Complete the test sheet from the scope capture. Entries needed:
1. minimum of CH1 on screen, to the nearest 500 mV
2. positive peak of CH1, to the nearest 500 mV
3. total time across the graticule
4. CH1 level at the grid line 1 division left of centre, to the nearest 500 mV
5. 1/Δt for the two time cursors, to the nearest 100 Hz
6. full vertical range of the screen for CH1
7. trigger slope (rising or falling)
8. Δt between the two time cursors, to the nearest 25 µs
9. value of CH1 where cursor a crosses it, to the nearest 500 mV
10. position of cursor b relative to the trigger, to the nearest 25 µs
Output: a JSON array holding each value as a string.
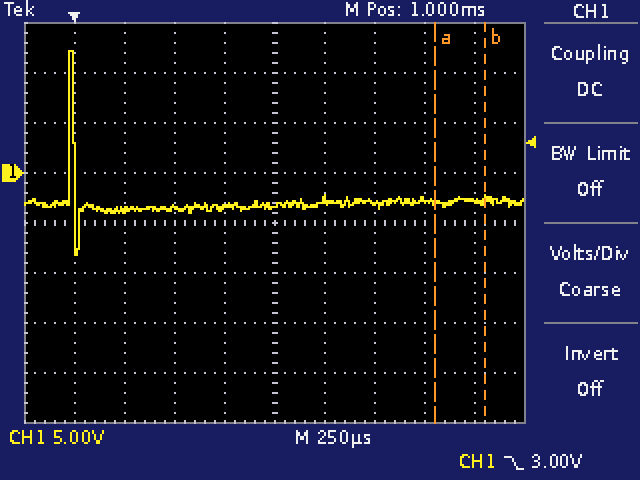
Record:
["-8.0 V", "12.0 V", "2.5 ms", "-3.5 V", "4.0 kHz", "40 V", "falling", "250 µs", "-3.0 V", "+2.050 ms"]
